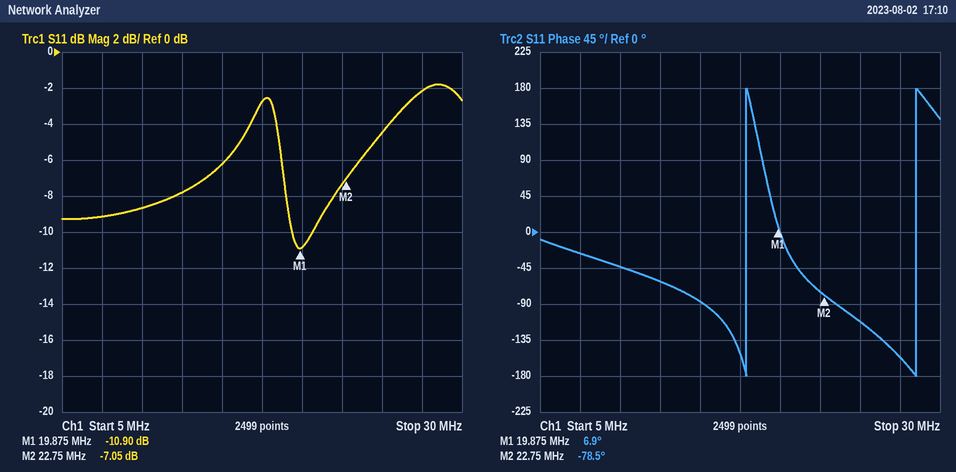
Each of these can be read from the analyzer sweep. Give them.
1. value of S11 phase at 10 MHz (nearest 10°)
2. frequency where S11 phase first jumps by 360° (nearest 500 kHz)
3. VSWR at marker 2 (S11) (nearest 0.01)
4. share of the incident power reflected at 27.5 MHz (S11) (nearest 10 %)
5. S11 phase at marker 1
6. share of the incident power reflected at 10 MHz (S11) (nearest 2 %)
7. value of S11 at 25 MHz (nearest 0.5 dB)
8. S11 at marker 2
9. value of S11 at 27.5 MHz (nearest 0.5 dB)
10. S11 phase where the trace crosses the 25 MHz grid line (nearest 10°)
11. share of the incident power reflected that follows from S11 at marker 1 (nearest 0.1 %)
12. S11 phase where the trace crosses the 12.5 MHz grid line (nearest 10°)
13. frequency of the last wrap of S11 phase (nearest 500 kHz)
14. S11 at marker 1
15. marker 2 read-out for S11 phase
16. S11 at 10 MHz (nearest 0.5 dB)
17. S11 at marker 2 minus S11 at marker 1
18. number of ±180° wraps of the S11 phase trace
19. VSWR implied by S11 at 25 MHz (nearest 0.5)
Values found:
-40°
18.0 MHz
2.60
60 %
6.9°
14 %
-4.5 dB
-7.05 dB
-2.0 dB
-110°
8.1 %
-60°
28.5 MHz
-10.90 dB
-78.5°
-8.5 dB
3.85 dB
2
4.0
